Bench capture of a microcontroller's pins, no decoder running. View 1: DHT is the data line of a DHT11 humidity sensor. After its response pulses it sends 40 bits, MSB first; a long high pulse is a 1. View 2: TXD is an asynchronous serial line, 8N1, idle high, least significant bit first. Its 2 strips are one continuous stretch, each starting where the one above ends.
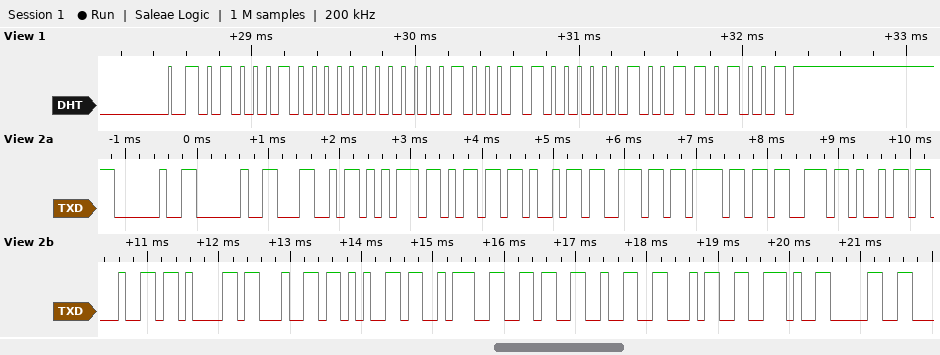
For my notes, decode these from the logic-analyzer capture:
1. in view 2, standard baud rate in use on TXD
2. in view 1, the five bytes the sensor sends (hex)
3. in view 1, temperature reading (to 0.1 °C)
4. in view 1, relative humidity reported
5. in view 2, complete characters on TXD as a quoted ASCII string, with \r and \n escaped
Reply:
9600 baud
44 00 23 02 69
35.2 °C
68 %
"  Luminosidade:624.0"
